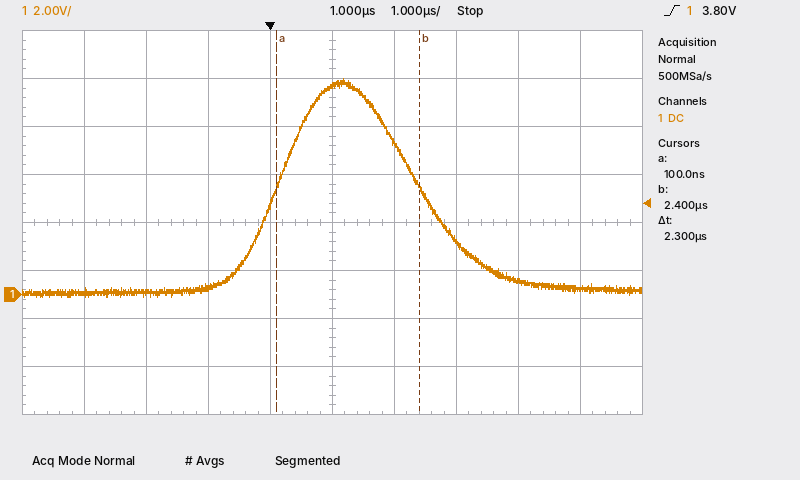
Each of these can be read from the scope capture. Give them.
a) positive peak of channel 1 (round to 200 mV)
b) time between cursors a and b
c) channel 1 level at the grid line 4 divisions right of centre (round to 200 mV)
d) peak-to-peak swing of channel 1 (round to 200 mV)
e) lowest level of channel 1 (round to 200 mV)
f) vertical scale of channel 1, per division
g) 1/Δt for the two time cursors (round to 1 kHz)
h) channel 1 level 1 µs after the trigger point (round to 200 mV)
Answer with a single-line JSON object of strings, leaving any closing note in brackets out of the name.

{"positive peak of channel 1": "9.0 V", "time between cursors a and b": "2.3 µs", "channel 1 level at the grid line 4 divisions right of centre": "200 mV", "peak-to-peak swing of channel 1": "9.2 V", "lowest level of channel 1": "-200 mV", "vertical scale of channel 1, per division": "2 V", "1/Δt for the two time cursors": "435 kHz", "channel 1 level 1 µs after the trigger point": "8.6 V"}
